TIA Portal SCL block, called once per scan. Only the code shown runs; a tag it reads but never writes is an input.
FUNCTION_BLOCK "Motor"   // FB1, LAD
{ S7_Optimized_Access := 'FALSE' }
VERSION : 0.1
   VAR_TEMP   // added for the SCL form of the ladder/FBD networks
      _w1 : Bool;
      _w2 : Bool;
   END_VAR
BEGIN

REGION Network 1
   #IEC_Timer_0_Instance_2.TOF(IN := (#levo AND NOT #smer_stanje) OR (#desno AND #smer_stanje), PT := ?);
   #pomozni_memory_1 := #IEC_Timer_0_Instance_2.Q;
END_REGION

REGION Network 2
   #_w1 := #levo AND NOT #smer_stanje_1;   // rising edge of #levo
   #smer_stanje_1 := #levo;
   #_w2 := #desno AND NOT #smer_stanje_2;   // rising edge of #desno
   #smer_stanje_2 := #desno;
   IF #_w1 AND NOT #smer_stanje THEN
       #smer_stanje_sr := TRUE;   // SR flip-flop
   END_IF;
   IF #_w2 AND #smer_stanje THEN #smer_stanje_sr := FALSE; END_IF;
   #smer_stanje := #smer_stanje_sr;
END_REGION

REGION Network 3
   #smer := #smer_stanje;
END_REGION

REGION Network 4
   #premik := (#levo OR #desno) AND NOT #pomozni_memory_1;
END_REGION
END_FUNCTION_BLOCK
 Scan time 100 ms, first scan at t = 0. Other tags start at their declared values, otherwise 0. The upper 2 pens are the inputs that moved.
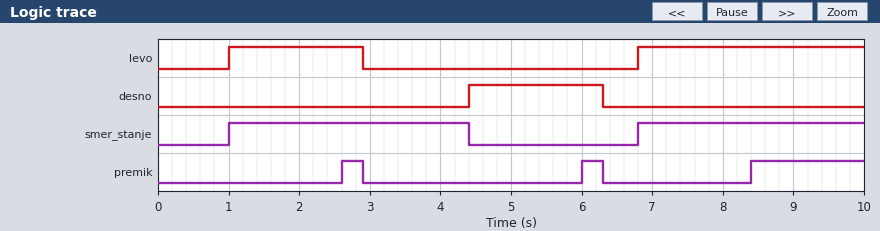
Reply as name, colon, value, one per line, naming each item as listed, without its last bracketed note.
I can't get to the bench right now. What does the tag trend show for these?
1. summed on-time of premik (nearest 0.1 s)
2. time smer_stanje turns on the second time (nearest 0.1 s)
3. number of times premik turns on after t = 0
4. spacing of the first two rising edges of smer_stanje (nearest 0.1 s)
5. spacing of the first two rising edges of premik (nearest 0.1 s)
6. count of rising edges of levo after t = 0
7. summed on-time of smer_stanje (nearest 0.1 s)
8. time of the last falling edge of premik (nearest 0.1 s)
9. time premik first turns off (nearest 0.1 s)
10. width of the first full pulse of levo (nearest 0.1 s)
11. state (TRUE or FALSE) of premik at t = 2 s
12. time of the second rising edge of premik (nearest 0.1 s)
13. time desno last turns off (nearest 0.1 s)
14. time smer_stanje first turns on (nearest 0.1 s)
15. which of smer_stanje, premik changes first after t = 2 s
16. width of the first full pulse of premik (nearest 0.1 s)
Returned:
summed on-time of premik: 2.2 s
time smer_stanje turns on the second time: 6.8 s
number of times premik turns on after t = 0: 3
spacing of the first two rising edges of smer_stanje: 5.8 s
spacing of the first two rising edges of premik: 3.4 s
count of rising edges of levo after t = 0: 2
summed on-time of smer_stanje: 6.6 s
time of the last falling edge of premik: 6.3 s
time premik first turns off: 2.9 s
width of the first full pulse of levo: 1.9 s
state (TRUE or FALSE) of premik at t = 2 s: FALSE
time of the second rising edge of premik: 6.0 s
time desno last turns off: 6.3 s
time smer_stanje first turns on: 1.0 s
which of smer_stanje, premik changes first after t = 2 s: premik
width of the first full pulse of premik: 0.3 s
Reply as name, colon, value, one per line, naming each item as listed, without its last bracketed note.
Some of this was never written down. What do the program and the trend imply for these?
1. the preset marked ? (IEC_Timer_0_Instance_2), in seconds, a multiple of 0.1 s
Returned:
the preset marked ? (IEC_Timer_0_Instance_2), in seconds, a multiple of 0.1 s: 1.5 s
